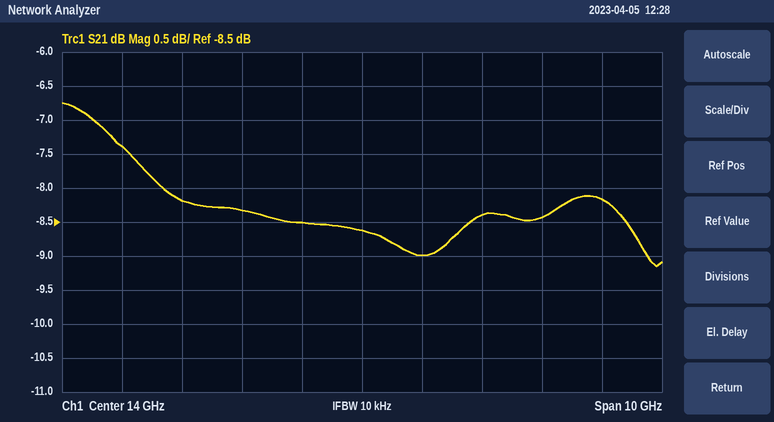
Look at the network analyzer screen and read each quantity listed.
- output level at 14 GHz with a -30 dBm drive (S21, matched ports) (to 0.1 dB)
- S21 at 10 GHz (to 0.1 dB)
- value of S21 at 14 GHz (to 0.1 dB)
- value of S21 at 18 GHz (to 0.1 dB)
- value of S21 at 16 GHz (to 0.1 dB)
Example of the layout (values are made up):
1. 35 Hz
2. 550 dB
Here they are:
1. -38.6 dBm
2. -7.4 dB
3. -8.6 dB
4. -8.2 dB
5. -8.4 dB
